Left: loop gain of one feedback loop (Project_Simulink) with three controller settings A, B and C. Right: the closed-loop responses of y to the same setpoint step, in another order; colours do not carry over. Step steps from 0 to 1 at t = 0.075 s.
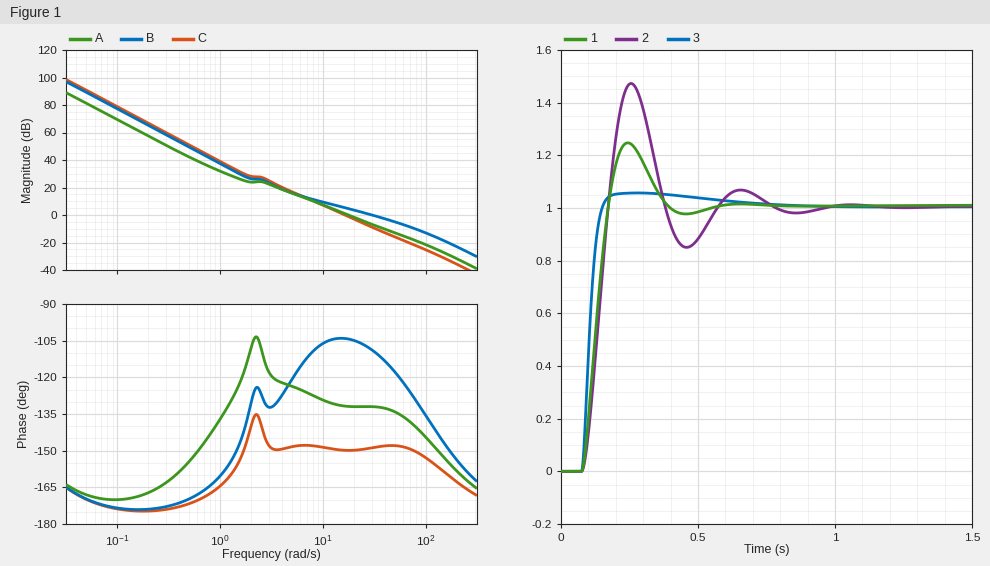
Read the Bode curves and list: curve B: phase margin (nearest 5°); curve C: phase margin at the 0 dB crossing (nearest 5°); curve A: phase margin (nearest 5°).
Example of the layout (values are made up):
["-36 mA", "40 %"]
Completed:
["70°", "30°", "50°"]
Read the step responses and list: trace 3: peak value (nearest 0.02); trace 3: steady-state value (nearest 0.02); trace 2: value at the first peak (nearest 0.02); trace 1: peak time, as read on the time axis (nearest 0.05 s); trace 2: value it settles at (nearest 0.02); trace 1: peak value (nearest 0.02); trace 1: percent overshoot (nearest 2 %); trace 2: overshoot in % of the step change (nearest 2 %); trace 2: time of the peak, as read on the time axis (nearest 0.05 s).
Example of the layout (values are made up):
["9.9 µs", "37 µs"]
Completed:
["1.06", "1.00", "1.48", "0.25 s", "1.00", "1.24", "24 %", "48 %", "0.25 s"]
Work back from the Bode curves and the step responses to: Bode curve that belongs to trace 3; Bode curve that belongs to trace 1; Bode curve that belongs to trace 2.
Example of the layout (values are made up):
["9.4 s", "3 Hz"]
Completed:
["B", "A", "C"]
